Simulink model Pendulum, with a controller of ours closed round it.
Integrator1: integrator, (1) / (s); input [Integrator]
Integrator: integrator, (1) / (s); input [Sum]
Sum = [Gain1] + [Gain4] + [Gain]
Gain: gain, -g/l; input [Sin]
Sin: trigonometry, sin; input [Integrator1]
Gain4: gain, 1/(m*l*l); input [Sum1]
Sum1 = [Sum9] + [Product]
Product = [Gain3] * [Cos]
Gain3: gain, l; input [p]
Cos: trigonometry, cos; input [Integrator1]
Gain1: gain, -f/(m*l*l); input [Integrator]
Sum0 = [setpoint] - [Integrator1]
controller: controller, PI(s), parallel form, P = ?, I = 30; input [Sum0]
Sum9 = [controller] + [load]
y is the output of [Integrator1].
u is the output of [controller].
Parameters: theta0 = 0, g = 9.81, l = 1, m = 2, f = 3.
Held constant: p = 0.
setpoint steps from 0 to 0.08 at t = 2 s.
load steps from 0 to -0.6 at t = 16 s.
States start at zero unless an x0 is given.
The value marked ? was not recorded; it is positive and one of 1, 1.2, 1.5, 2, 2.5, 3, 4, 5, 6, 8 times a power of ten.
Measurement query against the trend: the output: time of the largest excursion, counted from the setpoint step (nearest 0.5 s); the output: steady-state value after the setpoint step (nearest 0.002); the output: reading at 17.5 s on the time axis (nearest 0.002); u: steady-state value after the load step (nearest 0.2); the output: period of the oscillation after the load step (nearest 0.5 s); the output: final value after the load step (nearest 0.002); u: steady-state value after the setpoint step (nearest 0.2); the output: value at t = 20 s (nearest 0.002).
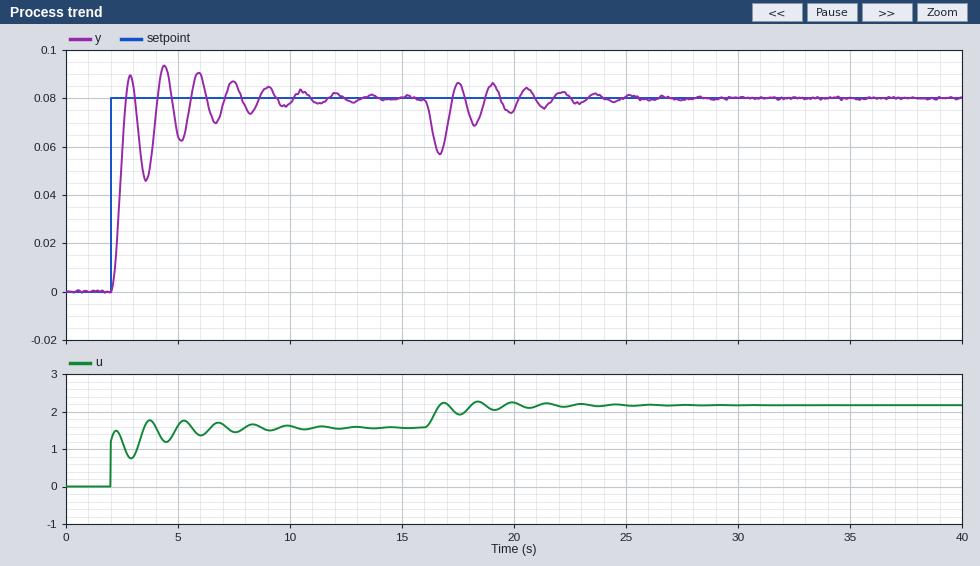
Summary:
2.5 s
0.080
0.086
2.2
1.5 s
0.080
1.6
0.076
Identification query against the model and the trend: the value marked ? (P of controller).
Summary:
15
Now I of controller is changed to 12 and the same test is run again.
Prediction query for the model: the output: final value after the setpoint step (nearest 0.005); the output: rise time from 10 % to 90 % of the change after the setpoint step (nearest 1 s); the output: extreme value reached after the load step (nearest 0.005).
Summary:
0.080
4 s
0.055
